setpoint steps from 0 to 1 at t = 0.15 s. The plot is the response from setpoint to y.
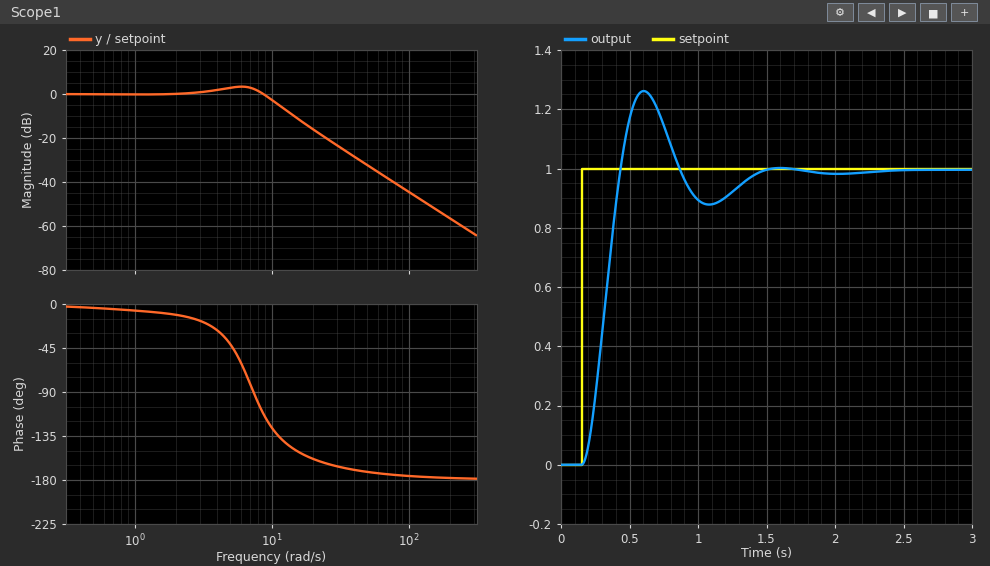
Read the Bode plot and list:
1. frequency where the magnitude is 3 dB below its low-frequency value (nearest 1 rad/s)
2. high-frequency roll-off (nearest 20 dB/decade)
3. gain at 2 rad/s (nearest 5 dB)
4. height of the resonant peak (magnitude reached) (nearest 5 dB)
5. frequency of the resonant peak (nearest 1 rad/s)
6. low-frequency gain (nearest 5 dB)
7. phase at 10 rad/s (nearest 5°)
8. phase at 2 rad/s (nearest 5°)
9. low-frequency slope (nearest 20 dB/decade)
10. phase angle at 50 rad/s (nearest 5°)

10 rad/s
-40 dB/decade
0 dB
5 dB
6 rad/s
0 dB
-125°
-10°
0 dB/decade
-170°
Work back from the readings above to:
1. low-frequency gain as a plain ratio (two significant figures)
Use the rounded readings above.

1.0
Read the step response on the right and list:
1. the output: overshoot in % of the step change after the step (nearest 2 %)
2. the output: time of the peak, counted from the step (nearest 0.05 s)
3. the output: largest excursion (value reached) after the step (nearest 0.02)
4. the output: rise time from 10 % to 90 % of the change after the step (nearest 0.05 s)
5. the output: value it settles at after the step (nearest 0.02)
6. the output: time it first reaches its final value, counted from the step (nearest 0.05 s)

26 %
0.45 s
1.26
0.20 s
1.00
0.30 s
